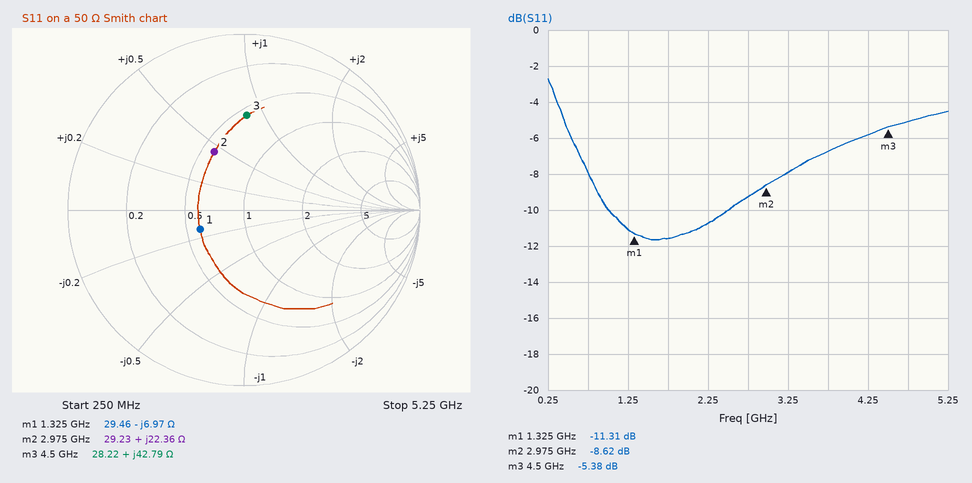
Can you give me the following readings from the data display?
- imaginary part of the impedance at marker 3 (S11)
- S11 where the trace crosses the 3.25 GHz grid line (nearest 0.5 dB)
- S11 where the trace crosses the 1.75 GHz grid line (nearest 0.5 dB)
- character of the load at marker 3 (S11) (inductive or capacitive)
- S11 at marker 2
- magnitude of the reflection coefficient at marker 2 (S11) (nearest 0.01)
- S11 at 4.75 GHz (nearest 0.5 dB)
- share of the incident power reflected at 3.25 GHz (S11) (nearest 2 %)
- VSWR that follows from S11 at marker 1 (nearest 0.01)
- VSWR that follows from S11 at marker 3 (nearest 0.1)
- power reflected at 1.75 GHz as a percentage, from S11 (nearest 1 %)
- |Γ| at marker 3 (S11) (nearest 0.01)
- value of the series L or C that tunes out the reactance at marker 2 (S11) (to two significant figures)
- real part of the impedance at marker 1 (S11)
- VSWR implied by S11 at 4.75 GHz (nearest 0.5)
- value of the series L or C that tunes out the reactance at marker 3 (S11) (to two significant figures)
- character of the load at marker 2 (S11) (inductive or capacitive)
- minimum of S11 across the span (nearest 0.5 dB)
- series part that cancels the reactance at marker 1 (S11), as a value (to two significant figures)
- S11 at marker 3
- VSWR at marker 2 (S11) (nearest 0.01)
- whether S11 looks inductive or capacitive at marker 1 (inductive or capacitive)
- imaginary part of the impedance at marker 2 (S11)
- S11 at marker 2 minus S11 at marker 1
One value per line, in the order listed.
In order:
+42.79 Ω
-8.0 dB
-11.5 dB
inductive
-8.62 dB
0.37
-5.0 dB
16 %
1.75
3.3
7 %
0.54
2.4 pF
29.46 Ω
3.5
830 fF
inductive
-11.5 dB
840 pH
-5.38 dB
2.18
capacitive
+22.36 Ω
2.69 dB
